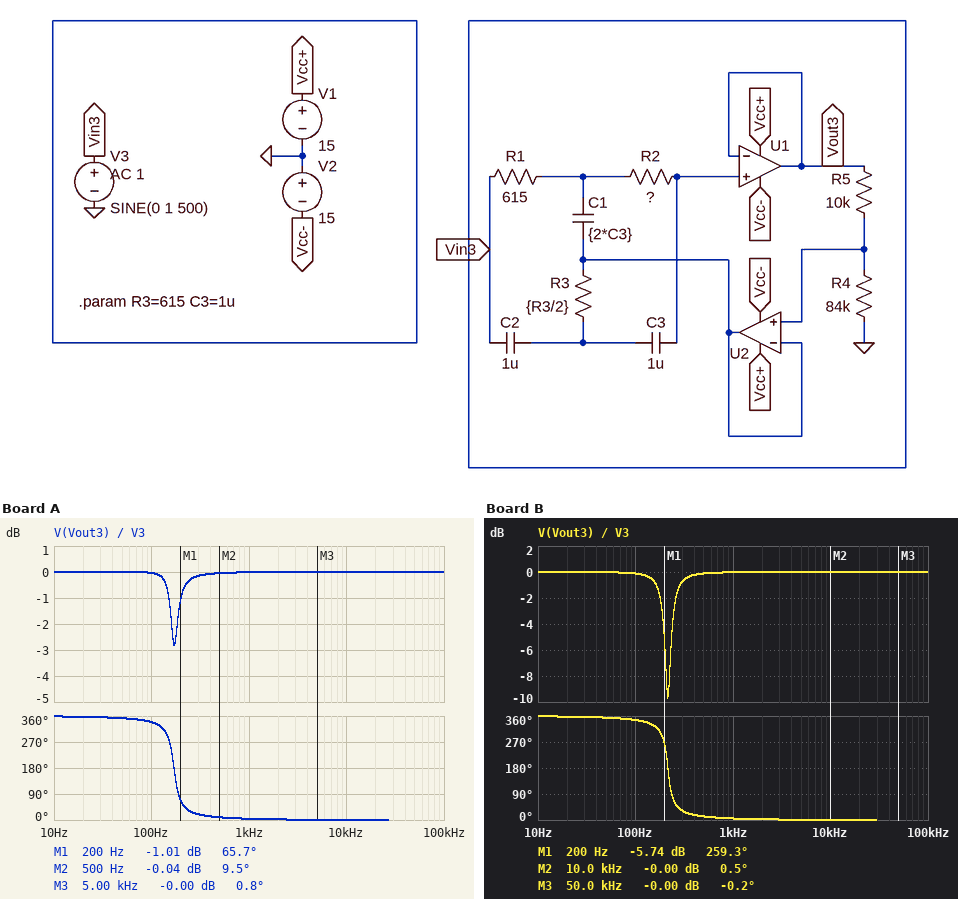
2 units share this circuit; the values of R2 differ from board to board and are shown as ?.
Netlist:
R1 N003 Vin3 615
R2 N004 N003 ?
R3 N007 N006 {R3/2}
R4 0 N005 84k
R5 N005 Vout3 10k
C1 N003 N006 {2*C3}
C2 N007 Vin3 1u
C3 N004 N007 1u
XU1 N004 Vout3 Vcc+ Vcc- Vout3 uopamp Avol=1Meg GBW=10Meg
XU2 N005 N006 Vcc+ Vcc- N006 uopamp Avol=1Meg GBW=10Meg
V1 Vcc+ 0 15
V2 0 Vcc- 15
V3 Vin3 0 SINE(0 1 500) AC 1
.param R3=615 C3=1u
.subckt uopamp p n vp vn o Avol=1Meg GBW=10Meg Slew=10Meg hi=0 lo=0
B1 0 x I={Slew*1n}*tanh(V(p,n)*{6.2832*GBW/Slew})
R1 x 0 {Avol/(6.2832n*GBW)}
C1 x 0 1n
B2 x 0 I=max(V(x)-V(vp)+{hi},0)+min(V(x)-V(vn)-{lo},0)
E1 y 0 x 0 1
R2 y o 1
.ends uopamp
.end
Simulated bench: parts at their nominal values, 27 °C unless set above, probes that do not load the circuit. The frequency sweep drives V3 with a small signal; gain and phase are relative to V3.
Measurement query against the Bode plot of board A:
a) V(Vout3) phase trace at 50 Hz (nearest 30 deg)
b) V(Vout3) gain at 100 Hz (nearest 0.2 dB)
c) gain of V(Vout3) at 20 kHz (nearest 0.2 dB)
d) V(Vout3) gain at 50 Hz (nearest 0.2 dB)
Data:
360 deg
0 dB
0 dB
0 dB
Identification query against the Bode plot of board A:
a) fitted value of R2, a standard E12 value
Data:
1.8 kΩ
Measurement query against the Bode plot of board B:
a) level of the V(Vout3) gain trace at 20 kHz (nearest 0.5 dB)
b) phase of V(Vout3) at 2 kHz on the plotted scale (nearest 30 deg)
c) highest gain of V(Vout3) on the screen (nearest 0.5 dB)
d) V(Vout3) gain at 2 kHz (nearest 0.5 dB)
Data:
0 dB
0 deg
0 dB
0 dB
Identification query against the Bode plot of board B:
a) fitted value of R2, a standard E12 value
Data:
1 kΩ
